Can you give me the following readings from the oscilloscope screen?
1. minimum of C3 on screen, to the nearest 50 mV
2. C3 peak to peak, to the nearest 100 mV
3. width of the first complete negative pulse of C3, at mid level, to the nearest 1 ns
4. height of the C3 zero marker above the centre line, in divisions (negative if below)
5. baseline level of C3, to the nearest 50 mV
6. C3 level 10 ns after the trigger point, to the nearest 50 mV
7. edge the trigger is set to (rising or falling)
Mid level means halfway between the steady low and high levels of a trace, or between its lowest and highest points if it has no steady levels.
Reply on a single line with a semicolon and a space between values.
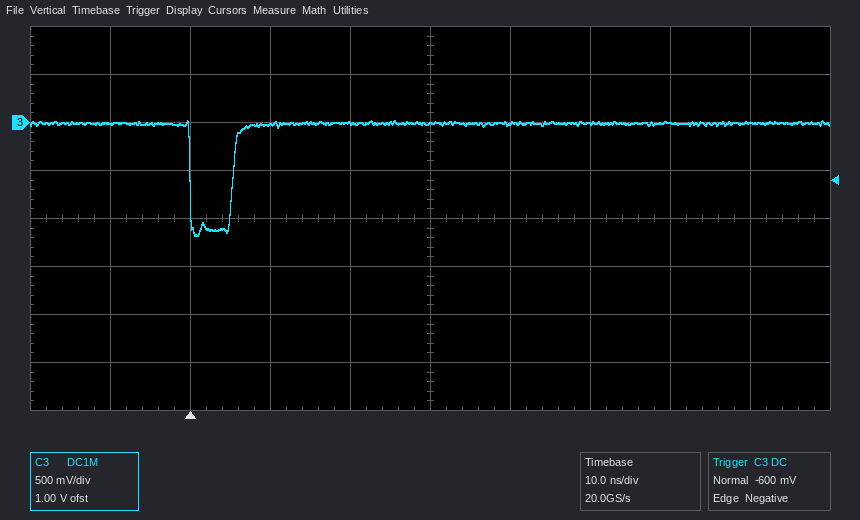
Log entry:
-1.20 V; 1.20 V; 5 ns; +2.0 div; 0 mV; 0 mV; falling
